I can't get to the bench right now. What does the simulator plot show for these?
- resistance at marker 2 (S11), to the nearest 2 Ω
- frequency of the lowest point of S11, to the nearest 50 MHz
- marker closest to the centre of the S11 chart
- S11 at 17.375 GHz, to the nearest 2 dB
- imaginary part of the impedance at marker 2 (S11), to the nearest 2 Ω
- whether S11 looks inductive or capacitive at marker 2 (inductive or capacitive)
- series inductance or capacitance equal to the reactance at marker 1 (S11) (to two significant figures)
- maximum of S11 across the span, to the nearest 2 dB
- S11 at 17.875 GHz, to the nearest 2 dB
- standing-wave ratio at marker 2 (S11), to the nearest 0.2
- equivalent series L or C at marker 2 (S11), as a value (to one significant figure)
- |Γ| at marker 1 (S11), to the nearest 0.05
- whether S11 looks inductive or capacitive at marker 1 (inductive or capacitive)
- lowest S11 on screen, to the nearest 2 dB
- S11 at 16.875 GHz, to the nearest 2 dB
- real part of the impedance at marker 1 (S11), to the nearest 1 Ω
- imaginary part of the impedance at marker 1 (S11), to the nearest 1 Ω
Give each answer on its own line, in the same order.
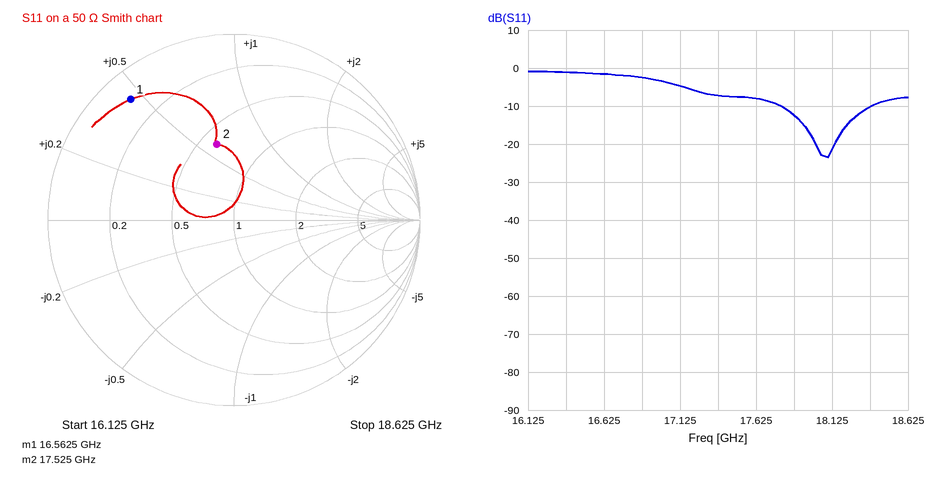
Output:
30 Ω
18.10 GHz
marker 2
-8 dB
+30 Ω
inductive
220 pH
0 dB
-12 dB
2.4
300 pH
0.85
inductive
-24 dB
-2 dB
5 Ω
+23 Ω
